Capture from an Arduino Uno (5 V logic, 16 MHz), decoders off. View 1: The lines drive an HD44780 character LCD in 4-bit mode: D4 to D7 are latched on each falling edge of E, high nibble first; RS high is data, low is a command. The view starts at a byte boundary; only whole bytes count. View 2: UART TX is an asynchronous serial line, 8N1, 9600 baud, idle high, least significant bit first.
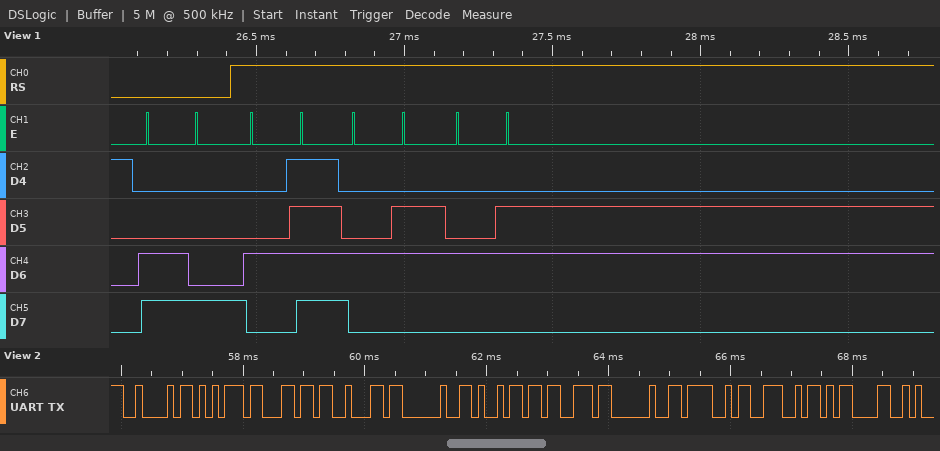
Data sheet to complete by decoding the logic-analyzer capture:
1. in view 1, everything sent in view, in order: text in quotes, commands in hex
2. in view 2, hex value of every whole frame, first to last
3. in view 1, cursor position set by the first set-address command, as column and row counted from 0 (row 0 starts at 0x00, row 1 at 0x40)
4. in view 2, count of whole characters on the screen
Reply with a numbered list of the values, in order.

1. 0xC8 "OFF"
2. 42 75 6C 62 20 69 73 20 4F 4E 0D
3. column 8, row 1
4. 11
